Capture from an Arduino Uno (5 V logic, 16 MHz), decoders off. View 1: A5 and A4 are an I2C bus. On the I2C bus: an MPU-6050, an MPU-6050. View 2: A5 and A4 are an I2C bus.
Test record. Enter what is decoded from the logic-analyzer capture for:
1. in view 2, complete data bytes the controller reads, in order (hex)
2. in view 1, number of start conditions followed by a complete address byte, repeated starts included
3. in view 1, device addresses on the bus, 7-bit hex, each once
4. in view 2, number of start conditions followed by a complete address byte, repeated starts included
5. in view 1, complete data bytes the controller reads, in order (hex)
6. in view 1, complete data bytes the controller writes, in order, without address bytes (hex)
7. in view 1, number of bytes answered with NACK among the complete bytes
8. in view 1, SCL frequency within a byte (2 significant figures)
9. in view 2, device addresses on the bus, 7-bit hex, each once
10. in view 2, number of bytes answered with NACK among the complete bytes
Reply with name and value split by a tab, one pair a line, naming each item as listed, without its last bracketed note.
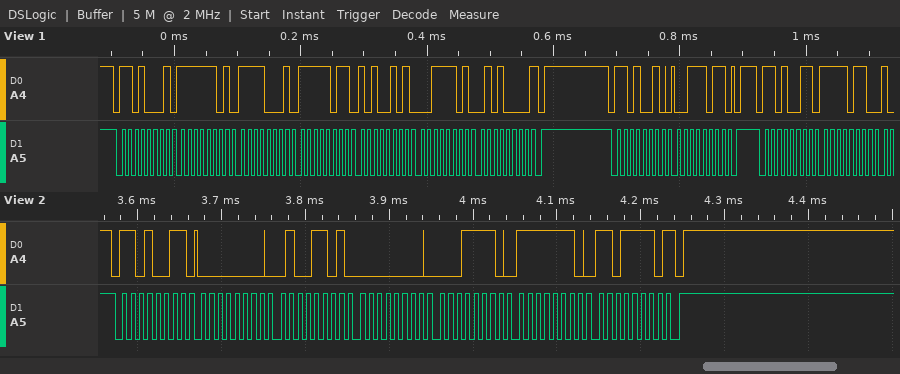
in view 2, complete data bytes the controller reads, in order	00 4D 00 1E FE DE
in view 1, number of start conditions followed by a complete address byte, repeated starts included	3
in view 1, device addresses on the bus, 7-bit hex, each once	0x68 0x69
in view 2, number of start conditions followed by a complete address byte, repeated starts included	1
in view 1, complete data bytes the controller reads, in order	FD F1 FB A5 3D 50 F6
in view 1, complete data bytes the controller writes, in order, without address bytes	3B
in view 1, number of bytes answered with NACK among the complete bytes	1
in view 1, SCL frequency within a byte	100 kHz
in view 2, device addresses on the bus, 7-bit hex, each once	0x69
in view 2, number of bytes answered with NACK among the complete bytes	1
